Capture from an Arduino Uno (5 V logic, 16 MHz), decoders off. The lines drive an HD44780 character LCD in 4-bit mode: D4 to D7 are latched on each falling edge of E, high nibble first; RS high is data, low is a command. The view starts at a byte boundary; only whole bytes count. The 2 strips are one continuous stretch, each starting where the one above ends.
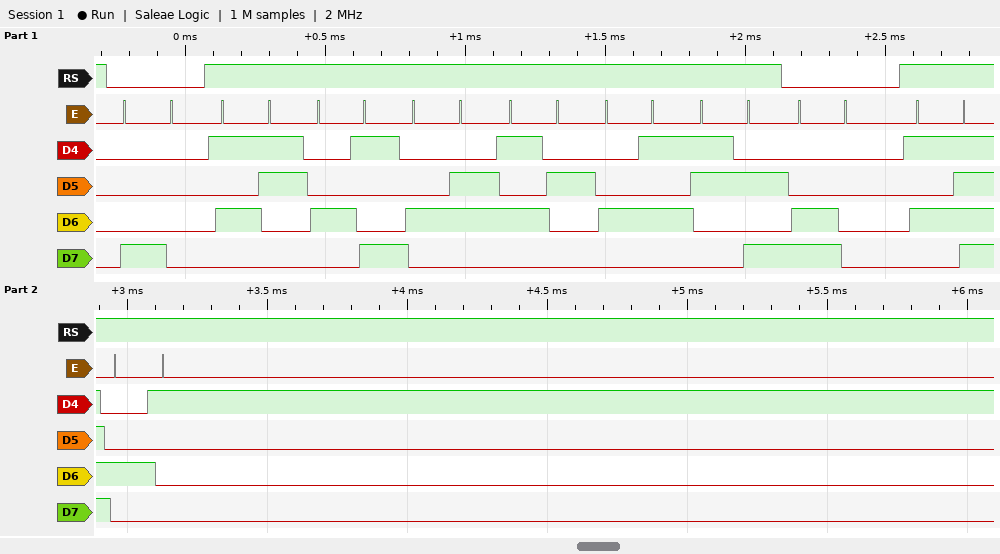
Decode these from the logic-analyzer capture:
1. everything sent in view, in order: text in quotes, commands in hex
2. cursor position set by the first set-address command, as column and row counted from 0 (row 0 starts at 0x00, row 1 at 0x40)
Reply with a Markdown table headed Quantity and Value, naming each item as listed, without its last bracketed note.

| Quantity | Value |
|---|---|
| everything sent in view, in order: text in quotes, commands in hex | 0x80 "SIFRE:" 0xC0 "_A" |
| cursor position set by the first set-address command, as column and row counted from 0 | column 0, row 0 |
